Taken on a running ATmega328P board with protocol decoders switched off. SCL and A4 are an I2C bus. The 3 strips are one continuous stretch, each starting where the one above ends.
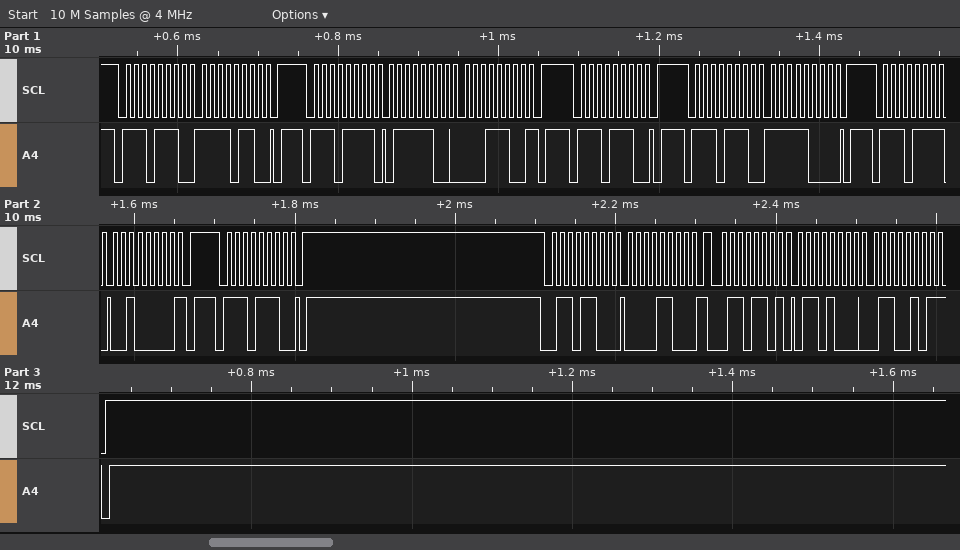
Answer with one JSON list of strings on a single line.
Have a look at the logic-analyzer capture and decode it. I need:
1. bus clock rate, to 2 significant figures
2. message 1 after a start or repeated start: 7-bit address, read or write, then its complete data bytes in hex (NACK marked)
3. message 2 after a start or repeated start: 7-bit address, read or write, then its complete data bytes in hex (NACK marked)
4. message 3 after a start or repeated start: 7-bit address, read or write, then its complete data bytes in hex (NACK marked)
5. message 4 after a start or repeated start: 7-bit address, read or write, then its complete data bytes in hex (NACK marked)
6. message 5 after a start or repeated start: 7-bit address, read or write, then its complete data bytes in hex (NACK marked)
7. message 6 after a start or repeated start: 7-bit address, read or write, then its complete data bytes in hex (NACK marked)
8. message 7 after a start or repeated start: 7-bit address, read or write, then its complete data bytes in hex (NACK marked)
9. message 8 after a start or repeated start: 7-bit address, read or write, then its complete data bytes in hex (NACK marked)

["100 kHz", "0x77 write: F6", "0x77 read: 7C 1C NACK", "0x77 write", "0x77 write: F8", "0x77 read: 20 NACK", "0x77 write", "0x36 write: 0C", "0x36 read: 68 65 NACK"]
